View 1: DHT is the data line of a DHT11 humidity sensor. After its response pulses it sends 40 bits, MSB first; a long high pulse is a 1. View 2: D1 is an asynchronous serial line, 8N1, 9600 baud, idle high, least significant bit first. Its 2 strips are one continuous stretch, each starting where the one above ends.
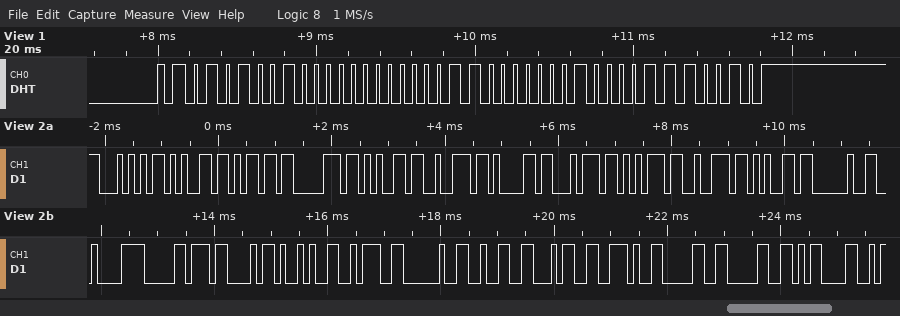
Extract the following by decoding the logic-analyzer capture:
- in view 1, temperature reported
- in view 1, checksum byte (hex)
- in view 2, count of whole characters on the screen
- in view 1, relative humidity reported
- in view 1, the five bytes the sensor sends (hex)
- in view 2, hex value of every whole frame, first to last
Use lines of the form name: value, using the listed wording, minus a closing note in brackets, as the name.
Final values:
in view 1, temperature reported: 24.8 °C
in view 1, checksum byte: 0x72
in view 2, count of whole characters on the screen: 24
in view 1, relative humidity reported: 82 %
in view 1, the five bytes the sensor sends: 52 00 18 08 72
in view 2, hex value of every whole frame, first to last: 54 65 6D 70 65 72 61 74 75 72 65 20 C2 B0 43 29 3A 20 32 34 2E 30 30 0D
